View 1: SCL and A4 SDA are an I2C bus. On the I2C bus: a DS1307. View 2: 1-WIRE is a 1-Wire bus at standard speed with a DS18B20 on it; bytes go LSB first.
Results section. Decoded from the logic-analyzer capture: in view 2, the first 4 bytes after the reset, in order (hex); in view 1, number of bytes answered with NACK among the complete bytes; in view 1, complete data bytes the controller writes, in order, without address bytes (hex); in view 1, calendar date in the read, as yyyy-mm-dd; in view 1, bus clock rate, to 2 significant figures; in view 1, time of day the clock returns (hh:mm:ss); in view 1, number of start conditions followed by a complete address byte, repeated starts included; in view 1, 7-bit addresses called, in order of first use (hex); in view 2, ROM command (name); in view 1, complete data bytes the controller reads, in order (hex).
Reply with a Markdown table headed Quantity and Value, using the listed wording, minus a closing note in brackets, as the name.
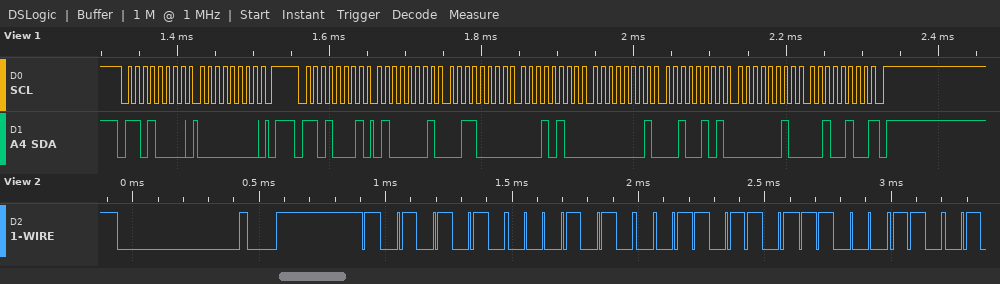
| Quantity | Value |
|---|---|
| in view 2, the first 4 bytes after the reset, in order | 55 28 B6 63 |
| in view 1, number of bytes answered with NACK among the complete bytes | 1 |
| in view 1, complete data bytes the controller writes, in order, without address bytes | 00 |
| in view 1, calendar date in the read, as yyyy-mm-dd | 2024-02-25 |
| in view 1, bus clock rate, to 2 significant figures | 100 kHz |
| in view 1, time of day the clock returns | 14:30:41 |
| in view 1, number of start conditions followed by a complete address byte, repeated starts included | 2 |
| in view 1, 7-bit addresses called, in order of first use | 0x68 |
| in view 2, ROM command | Match ROM |
| in view 1, complete data bytes the controller reads, in order | 41 30 14 01 25 02 24 |
